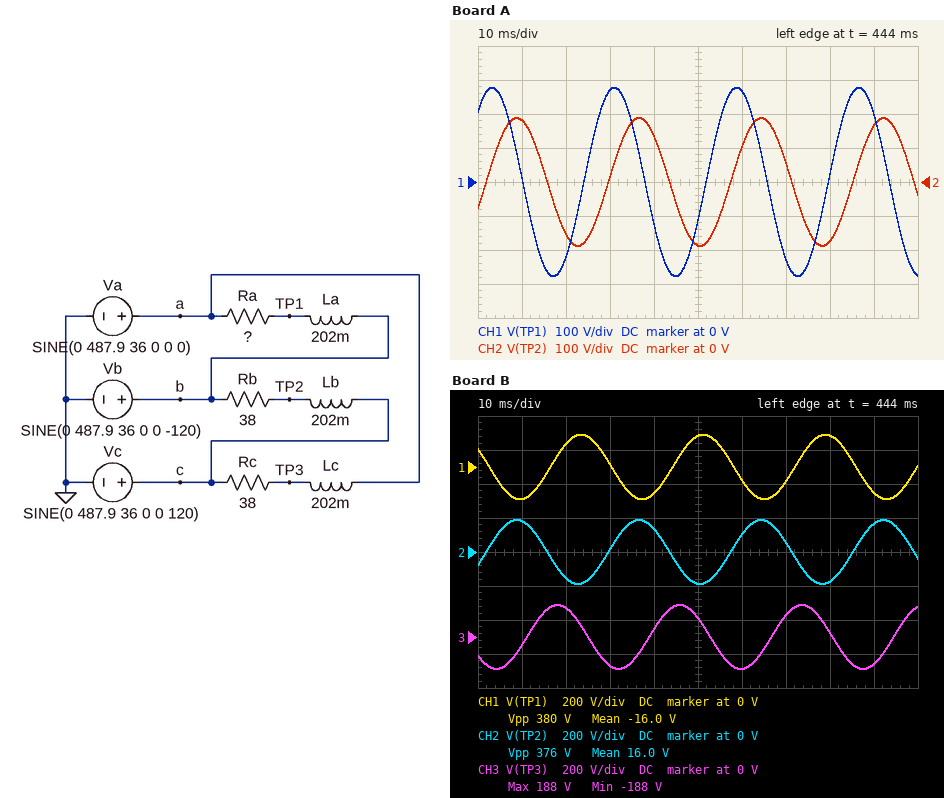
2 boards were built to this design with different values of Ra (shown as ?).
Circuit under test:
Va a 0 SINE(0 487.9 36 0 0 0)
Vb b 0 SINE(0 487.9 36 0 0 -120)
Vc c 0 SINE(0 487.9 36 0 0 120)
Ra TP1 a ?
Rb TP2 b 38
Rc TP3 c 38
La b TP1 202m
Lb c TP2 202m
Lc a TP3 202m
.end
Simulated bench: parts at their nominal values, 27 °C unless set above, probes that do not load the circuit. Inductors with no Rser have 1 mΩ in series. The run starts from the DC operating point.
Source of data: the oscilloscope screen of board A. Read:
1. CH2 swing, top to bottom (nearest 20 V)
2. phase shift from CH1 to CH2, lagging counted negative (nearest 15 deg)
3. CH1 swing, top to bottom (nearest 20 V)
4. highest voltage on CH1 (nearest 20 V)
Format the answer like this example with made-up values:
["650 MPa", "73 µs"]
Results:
["380 V", "-75 deg", "560 V", "280 V"]
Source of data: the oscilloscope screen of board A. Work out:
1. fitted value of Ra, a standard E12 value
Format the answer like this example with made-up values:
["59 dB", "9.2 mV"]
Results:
["22 Ω"]
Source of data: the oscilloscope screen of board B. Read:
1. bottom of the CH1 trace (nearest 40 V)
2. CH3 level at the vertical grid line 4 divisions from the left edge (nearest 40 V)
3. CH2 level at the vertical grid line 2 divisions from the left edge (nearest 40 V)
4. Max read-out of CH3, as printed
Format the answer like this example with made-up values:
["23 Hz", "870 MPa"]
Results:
["-200 V", "40 V", "-160 V", "188 V"]
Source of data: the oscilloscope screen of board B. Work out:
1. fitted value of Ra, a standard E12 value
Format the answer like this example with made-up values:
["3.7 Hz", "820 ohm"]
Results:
["56 Ω"]
